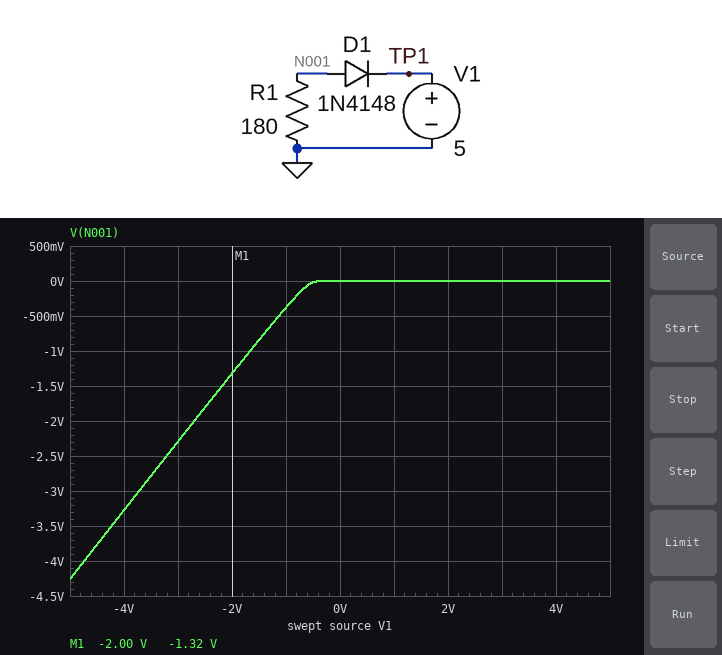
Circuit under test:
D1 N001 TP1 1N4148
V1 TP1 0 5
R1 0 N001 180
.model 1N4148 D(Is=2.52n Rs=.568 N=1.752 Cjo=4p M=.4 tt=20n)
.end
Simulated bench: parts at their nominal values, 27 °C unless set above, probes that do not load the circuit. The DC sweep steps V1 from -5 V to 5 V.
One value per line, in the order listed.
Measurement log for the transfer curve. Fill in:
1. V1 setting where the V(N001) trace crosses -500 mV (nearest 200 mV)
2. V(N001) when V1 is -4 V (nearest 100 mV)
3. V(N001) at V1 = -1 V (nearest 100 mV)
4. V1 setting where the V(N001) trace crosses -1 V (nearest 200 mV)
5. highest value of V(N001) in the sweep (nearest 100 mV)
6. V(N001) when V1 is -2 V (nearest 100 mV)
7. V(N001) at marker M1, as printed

-1.2 V
-3.3 V
-400 mV
-1.6 V
0 V
-1.3 V
-1.32 V
